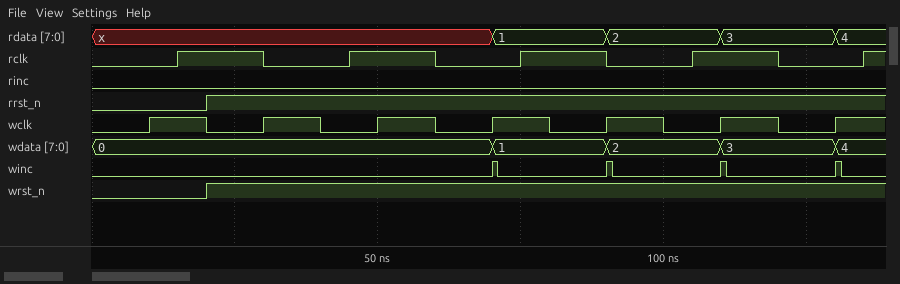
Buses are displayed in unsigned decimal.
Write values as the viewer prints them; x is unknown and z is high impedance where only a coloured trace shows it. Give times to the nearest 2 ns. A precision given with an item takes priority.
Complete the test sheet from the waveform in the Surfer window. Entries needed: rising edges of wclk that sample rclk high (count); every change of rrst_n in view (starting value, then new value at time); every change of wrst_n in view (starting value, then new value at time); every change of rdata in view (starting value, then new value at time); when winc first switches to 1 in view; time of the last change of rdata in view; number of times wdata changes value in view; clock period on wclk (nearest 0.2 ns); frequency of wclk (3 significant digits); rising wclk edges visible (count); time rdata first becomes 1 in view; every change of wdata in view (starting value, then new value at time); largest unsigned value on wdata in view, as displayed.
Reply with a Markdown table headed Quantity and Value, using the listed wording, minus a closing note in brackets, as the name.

| Quantity | Value |
|---|---|
| rising edges of wclk that sample rclk high | 4 |
| every change of rrst_n in view | 0, 1 at 20 ns |
| every change of wrst_n in view | 0, 1 at 20 ns |
| every change of rdata in view | x, 1 at 70 ns, 2 at 90 ns, 3 at 110 ns, 4 at 130 ns |
| when winc first switches to 1 in view | 70 ns |
| time of the last change of rdata in view | 130 ns |
| number of times wdata changes value in view | 4 |
| clock period on wclk | 20 ns |
| frequency of wclk | 50.0 MHz |
| rising wclk edges visible | 7 |
| time rdata first becomes 1 in view | 70 ns |
| every change of wdata in view | 0, 1 at 70 ns, 2 at 90 ns, 3 at 110 ns, 4 at 130 ns |
| largest unsigned value on wdata in view, as displayed | 4 |
